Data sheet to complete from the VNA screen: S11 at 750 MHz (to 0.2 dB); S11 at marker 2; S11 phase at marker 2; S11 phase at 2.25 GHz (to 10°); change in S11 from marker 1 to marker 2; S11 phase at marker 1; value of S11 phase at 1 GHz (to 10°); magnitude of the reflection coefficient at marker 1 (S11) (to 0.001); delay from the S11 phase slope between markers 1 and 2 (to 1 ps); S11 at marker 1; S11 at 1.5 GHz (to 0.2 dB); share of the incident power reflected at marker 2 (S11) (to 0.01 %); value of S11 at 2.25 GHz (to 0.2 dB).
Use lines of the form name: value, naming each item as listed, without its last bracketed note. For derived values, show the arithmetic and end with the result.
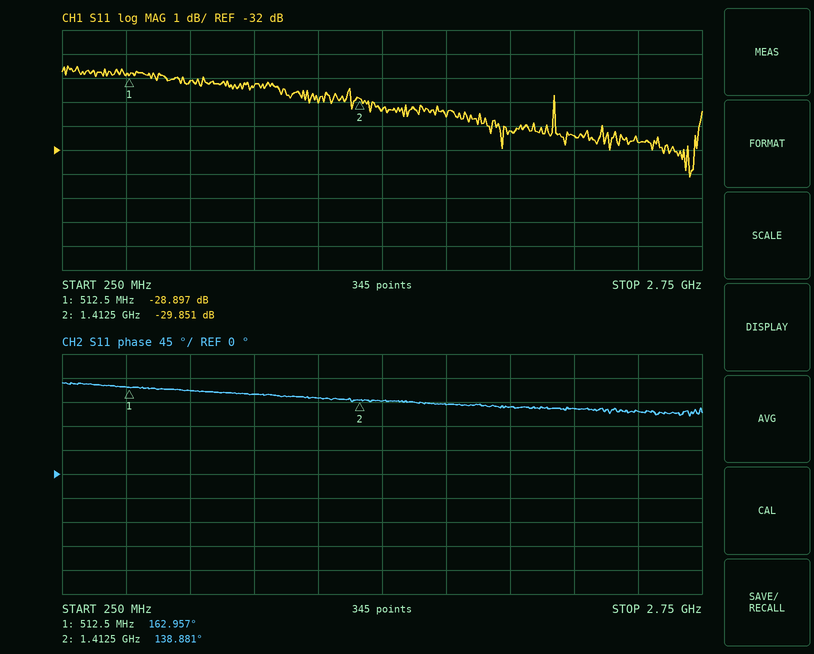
S11 at 750 MHz: -29.2 dB
S11 at marker 2: -29.851 dB
S11 phase at marker 2: 138.881°
S11 phase at 2.25 GHz: 120°
change in S11 from marker 1 to marker 2: -29.851 − (-28.897) = -0.954 dB
S11 phase at marker 1: 162.957°
value of S11 phase at 1 GHz: 150°
magnitude of the reflection coefficient at marker 1 (S11): 10^(-28.897/20) ≈ 0.036
delay from the S11 phase slope between markers 1 and 2: −(138.881° − (162.957°))/(360° × 900 MHz) ≈ 74 ps
S11 at marker 1: -28.897 dB
S11 at 1.5 GHz: -30.4 dB
share of the incident power reflected at marker 2 (S11): 10^(-29.851/10) ≈ 0.10 %
value of S11 at 2.25 GHz: -31.4 dB
